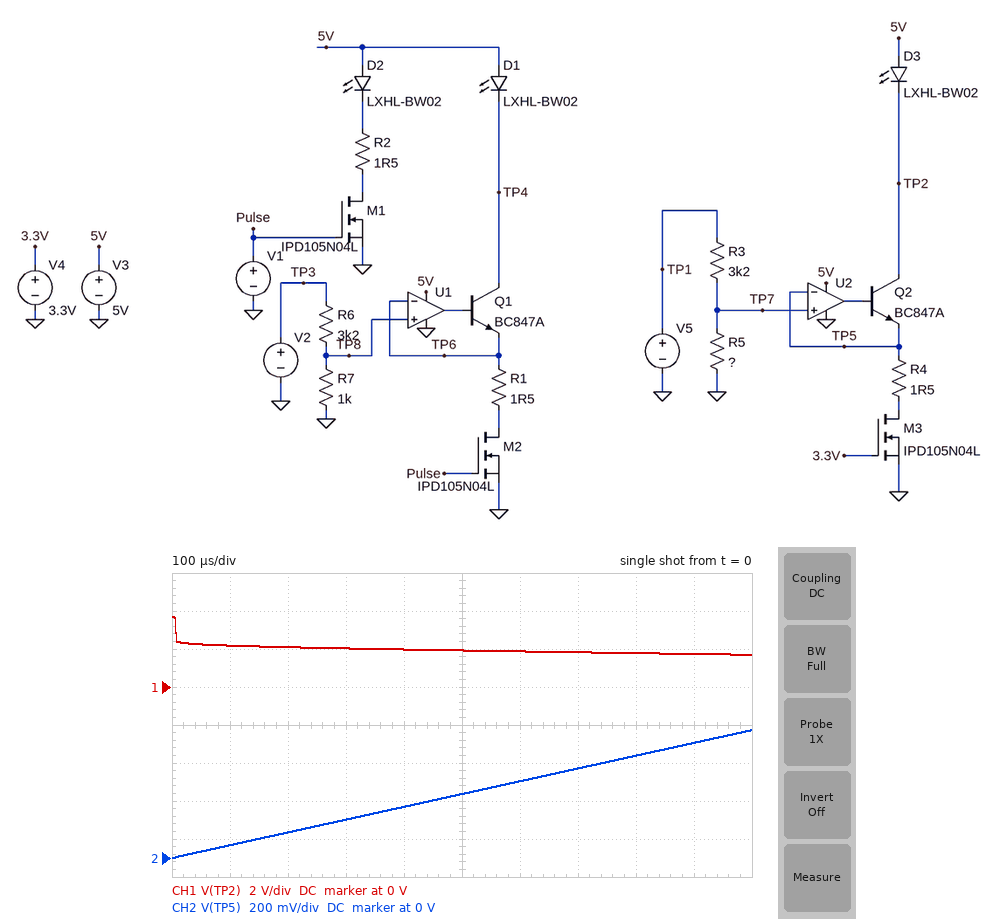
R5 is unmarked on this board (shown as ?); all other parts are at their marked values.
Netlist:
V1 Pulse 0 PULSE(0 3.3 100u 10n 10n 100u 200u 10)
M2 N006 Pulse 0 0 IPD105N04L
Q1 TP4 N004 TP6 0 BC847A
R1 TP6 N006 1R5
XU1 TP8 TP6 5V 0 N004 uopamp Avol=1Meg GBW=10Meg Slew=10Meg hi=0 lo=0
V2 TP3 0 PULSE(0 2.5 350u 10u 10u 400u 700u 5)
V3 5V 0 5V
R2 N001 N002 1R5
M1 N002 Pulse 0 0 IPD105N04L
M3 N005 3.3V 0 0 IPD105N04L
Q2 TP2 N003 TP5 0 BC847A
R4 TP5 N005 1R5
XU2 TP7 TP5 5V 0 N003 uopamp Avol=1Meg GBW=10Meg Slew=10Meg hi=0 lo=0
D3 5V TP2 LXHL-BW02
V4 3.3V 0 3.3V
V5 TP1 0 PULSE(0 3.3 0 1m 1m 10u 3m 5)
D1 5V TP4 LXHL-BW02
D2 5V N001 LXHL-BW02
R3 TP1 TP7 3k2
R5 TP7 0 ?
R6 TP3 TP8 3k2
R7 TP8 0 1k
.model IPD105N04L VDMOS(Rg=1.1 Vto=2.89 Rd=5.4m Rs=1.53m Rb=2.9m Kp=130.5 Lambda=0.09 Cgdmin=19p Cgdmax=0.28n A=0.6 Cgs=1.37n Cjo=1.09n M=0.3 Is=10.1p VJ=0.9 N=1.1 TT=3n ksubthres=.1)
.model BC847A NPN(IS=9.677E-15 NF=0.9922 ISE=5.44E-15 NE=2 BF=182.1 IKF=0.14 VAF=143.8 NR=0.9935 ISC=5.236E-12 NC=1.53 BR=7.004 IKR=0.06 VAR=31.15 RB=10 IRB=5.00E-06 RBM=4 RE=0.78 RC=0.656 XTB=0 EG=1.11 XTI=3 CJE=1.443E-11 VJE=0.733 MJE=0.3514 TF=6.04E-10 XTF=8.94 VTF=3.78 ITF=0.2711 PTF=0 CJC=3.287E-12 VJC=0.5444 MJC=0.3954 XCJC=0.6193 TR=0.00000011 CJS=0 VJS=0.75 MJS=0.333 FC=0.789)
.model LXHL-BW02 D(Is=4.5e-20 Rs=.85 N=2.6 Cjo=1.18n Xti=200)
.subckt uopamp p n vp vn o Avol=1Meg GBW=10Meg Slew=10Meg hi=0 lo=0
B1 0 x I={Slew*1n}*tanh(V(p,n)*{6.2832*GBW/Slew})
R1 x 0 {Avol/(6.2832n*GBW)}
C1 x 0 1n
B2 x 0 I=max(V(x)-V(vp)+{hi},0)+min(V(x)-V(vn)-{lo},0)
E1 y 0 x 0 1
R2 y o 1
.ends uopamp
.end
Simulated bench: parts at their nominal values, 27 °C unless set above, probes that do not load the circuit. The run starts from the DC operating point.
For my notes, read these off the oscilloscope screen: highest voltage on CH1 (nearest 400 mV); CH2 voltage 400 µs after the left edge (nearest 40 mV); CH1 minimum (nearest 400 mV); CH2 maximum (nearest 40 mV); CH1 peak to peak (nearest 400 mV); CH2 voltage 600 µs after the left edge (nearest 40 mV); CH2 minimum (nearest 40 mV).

3.6 V
280 mV
1.6 V
680 mV
2.0 V
400 mV
0 V
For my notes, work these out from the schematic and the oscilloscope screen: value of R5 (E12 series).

820 Ω
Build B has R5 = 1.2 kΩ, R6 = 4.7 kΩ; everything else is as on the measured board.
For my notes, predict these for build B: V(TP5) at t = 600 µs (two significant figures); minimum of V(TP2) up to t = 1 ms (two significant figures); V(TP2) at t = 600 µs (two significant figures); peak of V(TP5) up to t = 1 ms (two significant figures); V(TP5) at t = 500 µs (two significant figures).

540 mV
1.6 V
1.8 V
900 mV
450 mV
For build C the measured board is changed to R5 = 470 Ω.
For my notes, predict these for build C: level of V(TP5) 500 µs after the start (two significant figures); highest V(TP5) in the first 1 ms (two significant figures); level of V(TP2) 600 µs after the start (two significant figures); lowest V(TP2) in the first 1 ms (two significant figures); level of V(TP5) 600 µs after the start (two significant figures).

210 mV
420 mV
2.0 V
1.9 V
250 mV
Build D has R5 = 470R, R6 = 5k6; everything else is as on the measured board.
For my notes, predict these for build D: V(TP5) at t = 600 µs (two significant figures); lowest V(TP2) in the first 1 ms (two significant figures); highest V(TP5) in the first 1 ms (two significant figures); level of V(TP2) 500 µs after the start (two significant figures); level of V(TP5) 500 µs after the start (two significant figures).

250 mV
1.9 V
420 mV
2.0 V
210 mV
